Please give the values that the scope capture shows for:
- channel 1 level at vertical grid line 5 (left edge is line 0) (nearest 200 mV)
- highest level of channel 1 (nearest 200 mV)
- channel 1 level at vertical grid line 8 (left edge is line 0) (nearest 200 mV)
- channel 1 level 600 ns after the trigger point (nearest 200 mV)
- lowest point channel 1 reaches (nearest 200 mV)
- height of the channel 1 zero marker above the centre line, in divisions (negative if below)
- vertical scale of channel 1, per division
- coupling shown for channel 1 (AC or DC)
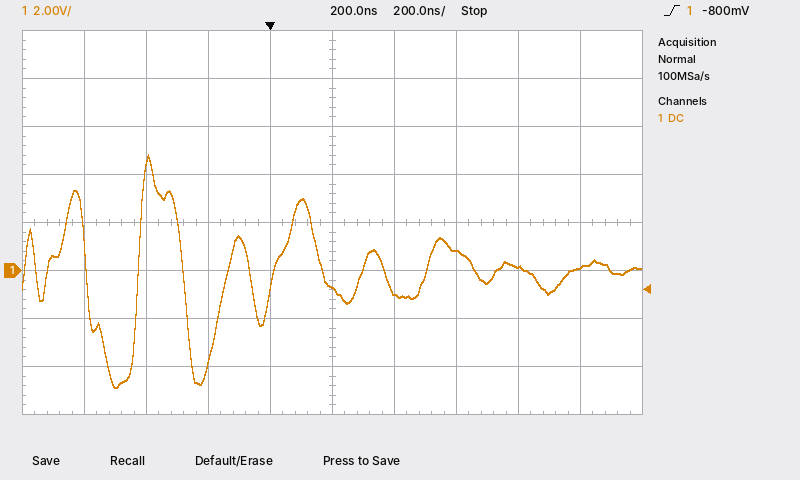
-800 mV
4.8 V
200 mV
800 mV
-4.8 V
-1.0 div
2 V
DC
